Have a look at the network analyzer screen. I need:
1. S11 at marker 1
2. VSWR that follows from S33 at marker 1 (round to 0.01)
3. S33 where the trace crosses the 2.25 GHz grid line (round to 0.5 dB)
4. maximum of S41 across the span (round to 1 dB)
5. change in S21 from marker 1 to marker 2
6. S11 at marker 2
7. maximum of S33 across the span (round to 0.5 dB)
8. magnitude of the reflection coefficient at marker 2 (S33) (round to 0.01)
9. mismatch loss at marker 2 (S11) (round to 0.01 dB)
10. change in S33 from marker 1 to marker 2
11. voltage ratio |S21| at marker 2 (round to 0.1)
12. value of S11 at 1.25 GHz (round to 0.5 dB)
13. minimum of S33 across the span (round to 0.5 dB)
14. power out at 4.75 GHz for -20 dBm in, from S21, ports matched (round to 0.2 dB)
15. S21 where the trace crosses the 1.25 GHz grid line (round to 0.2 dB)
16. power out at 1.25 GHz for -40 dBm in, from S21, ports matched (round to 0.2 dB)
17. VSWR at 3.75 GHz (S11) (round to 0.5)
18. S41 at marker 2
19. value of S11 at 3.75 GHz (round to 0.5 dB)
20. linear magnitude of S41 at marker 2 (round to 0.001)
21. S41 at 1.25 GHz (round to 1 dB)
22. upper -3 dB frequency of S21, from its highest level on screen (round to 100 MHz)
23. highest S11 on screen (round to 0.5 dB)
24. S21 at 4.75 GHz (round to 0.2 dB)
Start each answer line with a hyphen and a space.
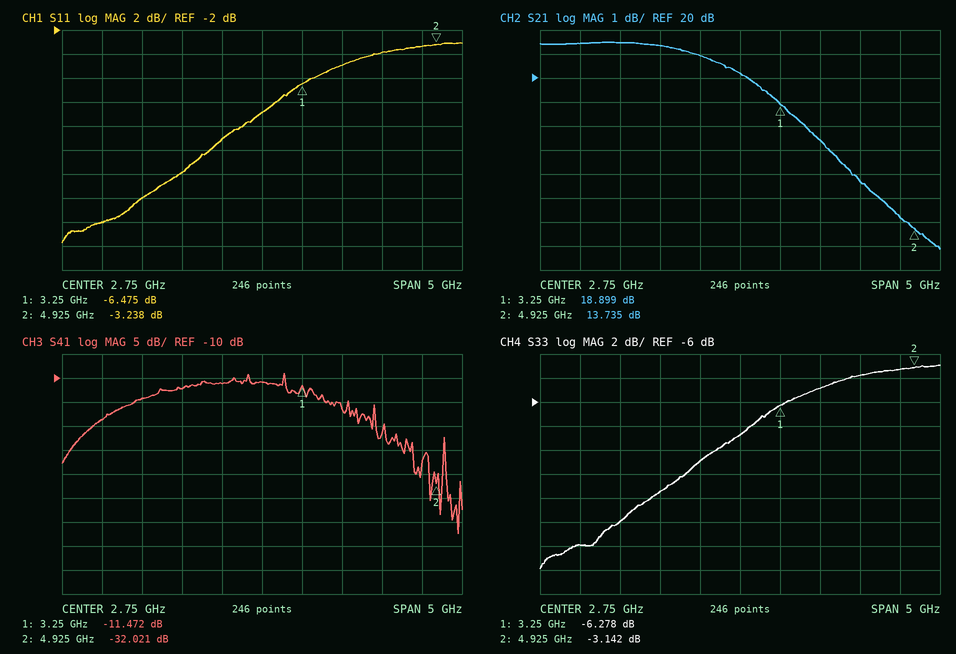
- -6.475 dB
- 2.89
- -11.0 dB
- -9 dB
- -5.164 dB
- -3.238 dB
- -3.0 dB
- 0.70
- 2.79 dB
- 3.136 dB
- 4.9
- -16.0 dB
- -20.0 dB
- -5.8 dBm
- 21.4 dB
- -18.6 dBm
- 3.5
- -32.021 dB
- -5.0 dB
- 0.025
- -14 dB
- 3.4 GHz
- -3.0 dB
- 14.2 dB
